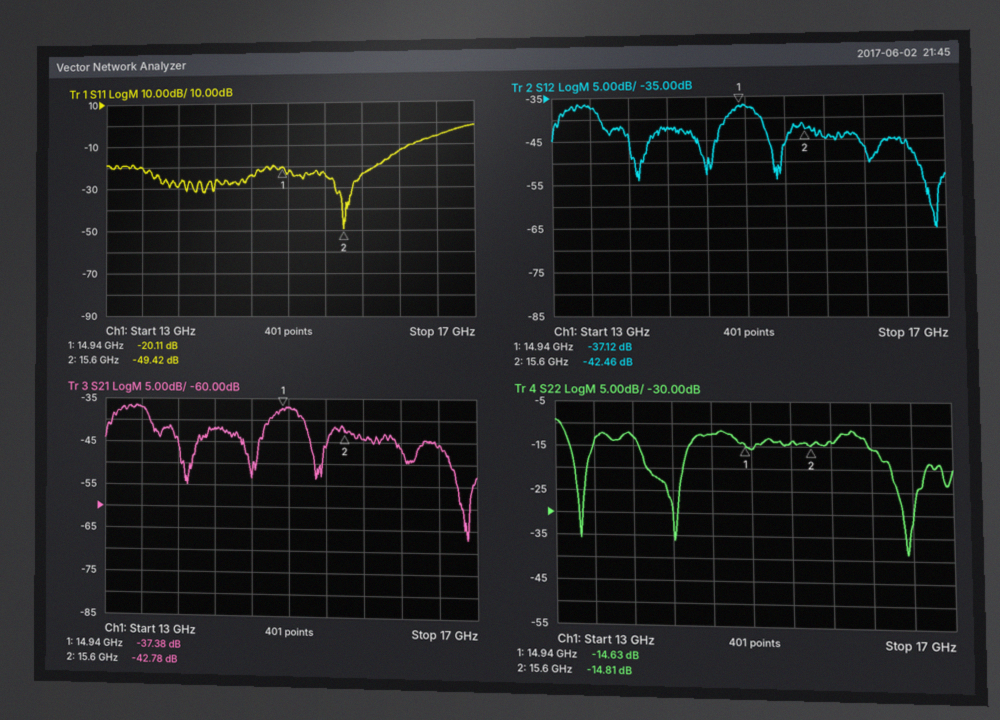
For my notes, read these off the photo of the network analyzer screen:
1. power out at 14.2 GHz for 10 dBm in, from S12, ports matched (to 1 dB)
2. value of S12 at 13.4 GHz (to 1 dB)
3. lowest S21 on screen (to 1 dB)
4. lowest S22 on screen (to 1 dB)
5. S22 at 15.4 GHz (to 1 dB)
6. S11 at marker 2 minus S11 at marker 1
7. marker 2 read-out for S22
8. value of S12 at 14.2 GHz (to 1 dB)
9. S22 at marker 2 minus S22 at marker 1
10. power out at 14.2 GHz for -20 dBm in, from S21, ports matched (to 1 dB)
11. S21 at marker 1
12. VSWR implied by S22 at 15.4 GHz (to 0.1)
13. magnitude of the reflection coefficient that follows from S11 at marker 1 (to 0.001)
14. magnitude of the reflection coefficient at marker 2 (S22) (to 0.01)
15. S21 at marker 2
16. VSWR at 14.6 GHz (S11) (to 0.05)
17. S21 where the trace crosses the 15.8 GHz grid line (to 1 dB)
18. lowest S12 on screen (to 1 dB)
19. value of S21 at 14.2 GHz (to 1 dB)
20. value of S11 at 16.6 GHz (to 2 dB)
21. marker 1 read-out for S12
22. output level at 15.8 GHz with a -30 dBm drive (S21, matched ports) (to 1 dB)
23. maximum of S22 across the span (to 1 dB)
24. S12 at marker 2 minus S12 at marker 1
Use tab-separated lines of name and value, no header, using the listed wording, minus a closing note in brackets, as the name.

power out at 14.2 GHz for 10 dBm in, from S12, ports matched	-32 dBm
value of S12 at 13.4 GHz	-37 dB
lowest S21 on screen	-67 dB
lowest S22 on screen	-39 dB
S22 at 15.4 GHz	-14 dB
S11 at marker 2 minus S11 at marker 1	-29.31 dB
marker 2 read-out for S22	-14.81 dB
value of S12 at 14.2 GHz	-42 dB
S22 at marker 2 minus S22 at marker 1	-0.18 dB
power out at 14.2 GHz for -20 dBm in, from S21, ports matched	-62 dBm
S21 at marker 1	-37.38 dB
VSWR implied by S22 at 15.4 GHz	1.5
magnitude of the reflection coefficient that follows from S11 at marker 1	0.099
magnitude of the reflection coefficient at marker 2 (S22)	0.18
S21 at marker 2	-42.78 dB
VSWR at 14.6 GHz (S11)	1.15
S21 where the trace crosses the 15.8 GHz grid line	-44 dB
lowest S12 on screen	-65 dB
value of S21 at 14.2 GHz	-42 dB
value of S11 at 16.6 GHz	-6 dB
marker 1 read-out for S12	-37.12 dB
output level at 15.8 GHz with a -30 dBm drive (S21, matched ports)	-74 dBm
maximum of S22 across the span	-9 dB
S12 at marker 2 minus S12 at marker 1	-5.34 dB
